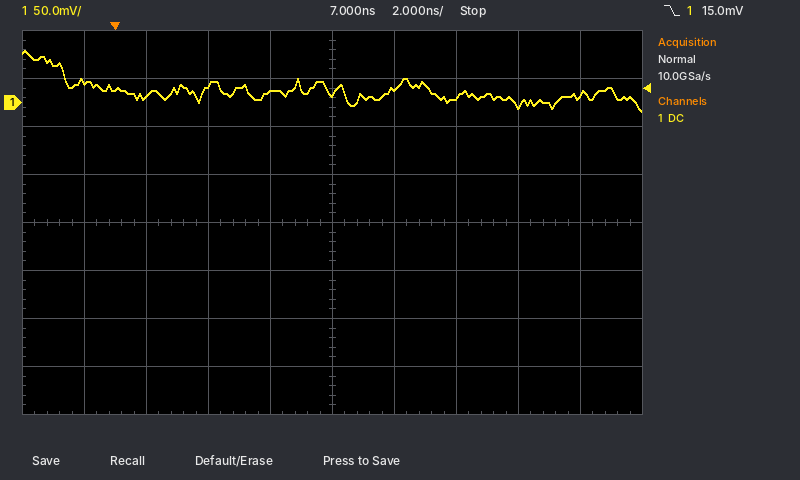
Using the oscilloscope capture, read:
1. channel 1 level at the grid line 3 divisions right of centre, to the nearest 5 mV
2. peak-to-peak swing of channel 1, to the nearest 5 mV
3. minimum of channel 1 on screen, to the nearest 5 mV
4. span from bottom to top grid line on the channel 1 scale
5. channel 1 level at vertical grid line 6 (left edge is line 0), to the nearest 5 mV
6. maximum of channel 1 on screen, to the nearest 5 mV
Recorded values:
-5 mV
65 mV
-10 mV
400 mV
15 mV
55 mV
